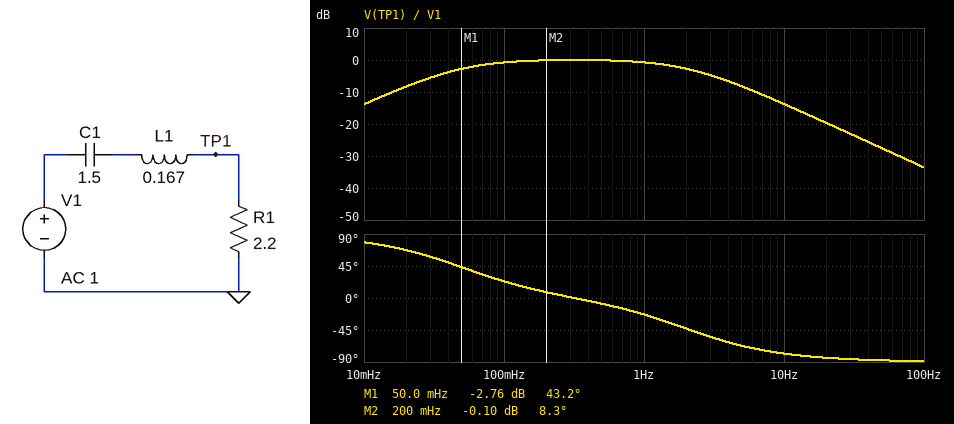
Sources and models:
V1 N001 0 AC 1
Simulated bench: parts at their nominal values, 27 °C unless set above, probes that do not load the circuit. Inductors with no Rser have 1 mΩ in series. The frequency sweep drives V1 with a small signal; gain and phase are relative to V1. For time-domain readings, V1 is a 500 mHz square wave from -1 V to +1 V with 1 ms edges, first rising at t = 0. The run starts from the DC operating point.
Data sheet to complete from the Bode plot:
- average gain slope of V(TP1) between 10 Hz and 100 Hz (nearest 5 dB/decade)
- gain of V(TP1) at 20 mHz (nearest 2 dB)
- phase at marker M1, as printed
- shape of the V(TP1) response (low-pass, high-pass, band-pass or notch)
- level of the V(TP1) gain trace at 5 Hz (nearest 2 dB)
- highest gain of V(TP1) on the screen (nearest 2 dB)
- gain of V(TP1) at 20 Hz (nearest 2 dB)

-20 dB/decade
-8 dB
43.2 deg
band-pass
-8 dB
0 dB
-20 dB
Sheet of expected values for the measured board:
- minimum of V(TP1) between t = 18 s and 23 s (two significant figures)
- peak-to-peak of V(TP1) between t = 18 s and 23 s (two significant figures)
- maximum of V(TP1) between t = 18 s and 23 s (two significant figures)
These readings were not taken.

-1.1 V
2.1 V
1.1 V
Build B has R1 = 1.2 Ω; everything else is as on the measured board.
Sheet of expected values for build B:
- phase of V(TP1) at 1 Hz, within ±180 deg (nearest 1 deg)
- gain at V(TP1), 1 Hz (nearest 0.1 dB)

-38 deg
-2.1 dB
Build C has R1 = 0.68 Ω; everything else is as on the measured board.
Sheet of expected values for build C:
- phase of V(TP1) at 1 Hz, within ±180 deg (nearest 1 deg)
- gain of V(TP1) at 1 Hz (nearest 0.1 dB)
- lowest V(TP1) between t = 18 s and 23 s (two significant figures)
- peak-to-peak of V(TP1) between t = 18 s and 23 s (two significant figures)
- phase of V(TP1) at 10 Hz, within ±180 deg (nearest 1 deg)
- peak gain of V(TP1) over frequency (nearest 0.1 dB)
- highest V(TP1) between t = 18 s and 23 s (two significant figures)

-54 deg
-4.7 dB
-1.0 V
2.0 V
-86 deg
0 dB
1.0 V
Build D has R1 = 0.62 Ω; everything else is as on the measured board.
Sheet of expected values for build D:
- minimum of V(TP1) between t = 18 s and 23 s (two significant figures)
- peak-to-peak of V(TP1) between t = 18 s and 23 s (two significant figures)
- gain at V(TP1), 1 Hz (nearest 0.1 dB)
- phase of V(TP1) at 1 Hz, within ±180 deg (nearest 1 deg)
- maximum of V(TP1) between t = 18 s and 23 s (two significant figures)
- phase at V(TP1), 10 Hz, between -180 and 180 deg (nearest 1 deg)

-1.0 V
2.0 V
-5.2 dB
-57 deg
1.0 V
-87 deg
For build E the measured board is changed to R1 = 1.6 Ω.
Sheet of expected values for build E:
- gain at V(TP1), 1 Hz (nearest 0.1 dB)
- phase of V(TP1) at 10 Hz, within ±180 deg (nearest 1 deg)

-1.3 dB
-81 deg
